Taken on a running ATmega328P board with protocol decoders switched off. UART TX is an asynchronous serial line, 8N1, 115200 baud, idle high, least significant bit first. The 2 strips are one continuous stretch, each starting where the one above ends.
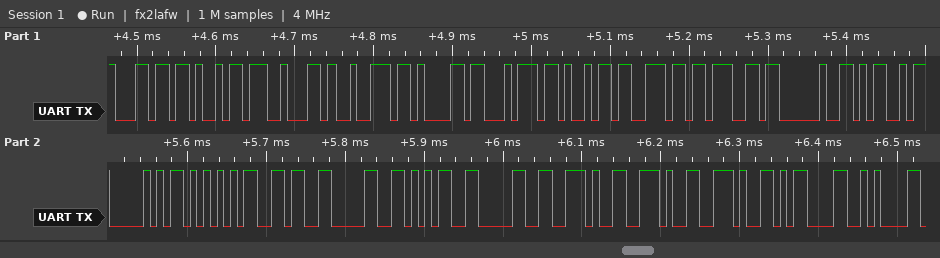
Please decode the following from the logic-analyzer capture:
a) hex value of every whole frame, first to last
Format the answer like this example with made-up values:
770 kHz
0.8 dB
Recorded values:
0x6C 0x69 0x62 0x72 0x61 0x74 0x69 0x6E 0x67 0x20 0x4D 0x50 0x55 0x36 0x30 0x35 0x30 0x2E 0x2E 0x2E 0x0D 0x0A
